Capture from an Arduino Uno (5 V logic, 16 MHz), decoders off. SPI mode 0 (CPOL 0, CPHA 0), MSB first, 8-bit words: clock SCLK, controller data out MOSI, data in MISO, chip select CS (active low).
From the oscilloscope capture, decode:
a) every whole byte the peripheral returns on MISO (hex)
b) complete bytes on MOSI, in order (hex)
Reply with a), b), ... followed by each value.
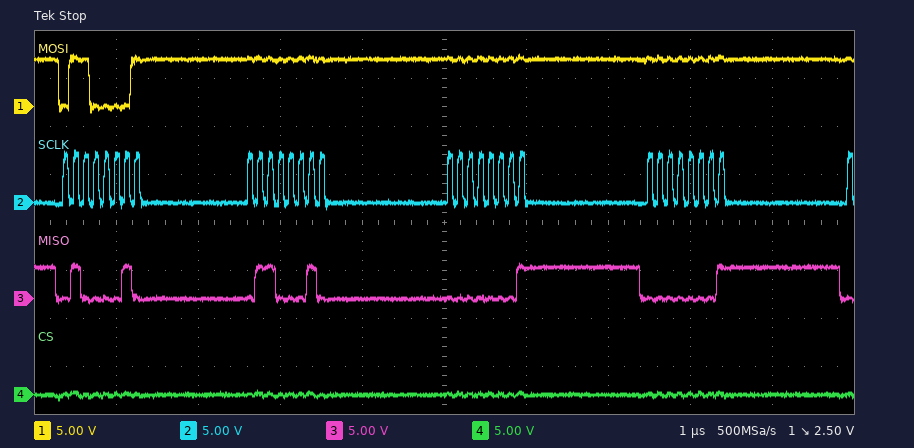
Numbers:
a) 42 62 01 01
b) 61 FF FF FF
